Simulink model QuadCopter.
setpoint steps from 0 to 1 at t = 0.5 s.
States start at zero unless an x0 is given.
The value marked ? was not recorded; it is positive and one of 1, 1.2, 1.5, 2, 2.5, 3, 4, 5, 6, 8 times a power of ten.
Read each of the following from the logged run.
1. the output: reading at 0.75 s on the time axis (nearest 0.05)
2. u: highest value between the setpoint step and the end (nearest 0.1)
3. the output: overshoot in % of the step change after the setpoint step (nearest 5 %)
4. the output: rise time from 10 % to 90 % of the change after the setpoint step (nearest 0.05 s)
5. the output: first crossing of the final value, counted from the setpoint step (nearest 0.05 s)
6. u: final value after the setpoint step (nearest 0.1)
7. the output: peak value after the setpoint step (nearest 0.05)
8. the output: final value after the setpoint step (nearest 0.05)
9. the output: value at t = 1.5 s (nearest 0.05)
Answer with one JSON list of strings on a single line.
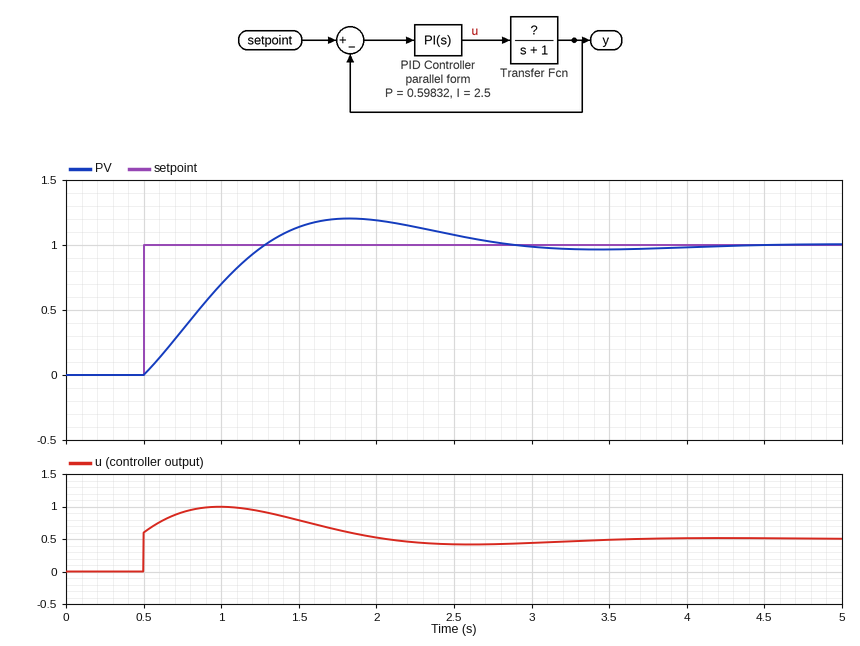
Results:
["0.35", "1.0", "20 %", "0.60 s", "0.80 s", "0.5", "1.20", "1.00", "1.15"]
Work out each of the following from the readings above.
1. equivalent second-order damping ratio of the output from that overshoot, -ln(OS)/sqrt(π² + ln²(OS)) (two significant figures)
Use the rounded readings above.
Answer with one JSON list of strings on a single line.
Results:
["0.46"]
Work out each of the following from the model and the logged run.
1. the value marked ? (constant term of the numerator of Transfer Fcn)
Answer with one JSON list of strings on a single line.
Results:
["2"]
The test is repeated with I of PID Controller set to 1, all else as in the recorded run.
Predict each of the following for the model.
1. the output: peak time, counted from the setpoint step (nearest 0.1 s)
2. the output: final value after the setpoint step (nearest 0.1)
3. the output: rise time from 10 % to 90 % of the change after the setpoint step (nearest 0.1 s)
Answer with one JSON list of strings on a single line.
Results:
["2.4 s", "1.0", "1.1 s"]
